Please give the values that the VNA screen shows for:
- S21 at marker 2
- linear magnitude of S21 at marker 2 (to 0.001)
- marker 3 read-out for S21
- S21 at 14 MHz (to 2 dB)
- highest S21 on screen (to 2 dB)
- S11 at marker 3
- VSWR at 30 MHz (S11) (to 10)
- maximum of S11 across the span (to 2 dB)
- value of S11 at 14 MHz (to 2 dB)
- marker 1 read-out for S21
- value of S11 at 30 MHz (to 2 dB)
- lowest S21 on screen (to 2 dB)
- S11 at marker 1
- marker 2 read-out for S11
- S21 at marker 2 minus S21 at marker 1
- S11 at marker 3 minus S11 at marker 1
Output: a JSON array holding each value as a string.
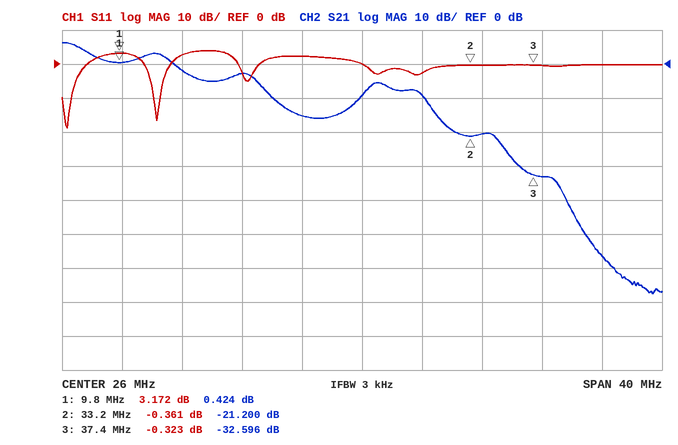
["-21.200 dB", "0.087", "-32.596 dB", "-2 dB", "6 dB", "-0.323 dB", "10", "4 dB", "2 dB", "0.424 dB", "-2 dB", "-68 dB", "3.172 dB", "-0.361 dB", "-21.624 dB", "-3.495 dB"]
